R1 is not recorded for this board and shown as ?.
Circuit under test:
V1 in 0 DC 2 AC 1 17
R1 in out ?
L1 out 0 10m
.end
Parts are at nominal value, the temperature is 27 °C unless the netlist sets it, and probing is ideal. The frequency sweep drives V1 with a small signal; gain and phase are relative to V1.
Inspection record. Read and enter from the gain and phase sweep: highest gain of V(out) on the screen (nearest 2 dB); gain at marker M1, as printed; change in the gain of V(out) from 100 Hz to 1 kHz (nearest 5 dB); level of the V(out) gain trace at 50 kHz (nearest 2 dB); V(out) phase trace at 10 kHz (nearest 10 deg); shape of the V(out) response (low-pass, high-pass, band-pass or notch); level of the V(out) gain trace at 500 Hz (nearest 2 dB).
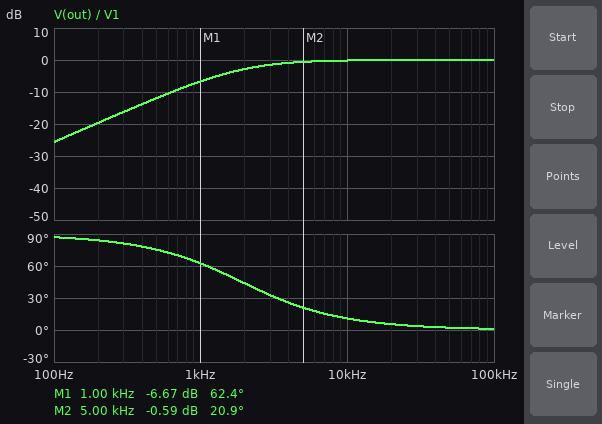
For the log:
0 dB
-6.67 dB
20 dB
0 dB
10 deg
high-pass
-12 dB
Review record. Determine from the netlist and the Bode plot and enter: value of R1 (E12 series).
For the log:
120 Ω
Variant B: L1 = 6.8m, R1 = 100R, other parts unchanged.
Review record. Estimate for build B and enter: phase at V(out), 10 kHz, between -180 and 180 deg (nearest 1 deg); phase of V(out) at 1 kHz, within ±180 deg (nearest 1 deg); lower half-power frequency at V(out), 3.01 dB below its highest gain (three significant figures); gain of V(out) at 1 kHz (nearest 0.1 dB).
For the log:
13 deg
67 deg
2.34 kHz
-8.1 dB
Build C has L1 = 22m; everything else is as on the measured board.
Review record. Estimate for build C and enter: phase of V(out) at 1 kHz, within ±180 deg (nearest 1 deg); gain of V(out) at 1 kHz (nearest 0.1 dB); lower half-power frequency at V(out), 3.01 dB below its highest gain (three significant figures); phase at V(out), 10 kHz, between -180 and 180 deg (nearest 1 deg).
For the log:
41 deg
-2.4 dB
868 Hz
5 deg
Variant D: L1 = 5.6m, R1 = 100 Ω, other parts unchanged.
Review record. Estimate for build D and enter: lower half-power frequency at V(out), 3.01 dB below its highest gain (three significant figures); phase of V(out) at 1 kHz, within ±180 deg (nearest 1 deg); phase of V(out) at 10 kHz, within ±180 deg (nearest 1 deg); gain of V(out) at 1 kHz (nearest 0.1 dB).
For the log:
2.84 kHz
71 deg
16 deg
-9.6 dB
